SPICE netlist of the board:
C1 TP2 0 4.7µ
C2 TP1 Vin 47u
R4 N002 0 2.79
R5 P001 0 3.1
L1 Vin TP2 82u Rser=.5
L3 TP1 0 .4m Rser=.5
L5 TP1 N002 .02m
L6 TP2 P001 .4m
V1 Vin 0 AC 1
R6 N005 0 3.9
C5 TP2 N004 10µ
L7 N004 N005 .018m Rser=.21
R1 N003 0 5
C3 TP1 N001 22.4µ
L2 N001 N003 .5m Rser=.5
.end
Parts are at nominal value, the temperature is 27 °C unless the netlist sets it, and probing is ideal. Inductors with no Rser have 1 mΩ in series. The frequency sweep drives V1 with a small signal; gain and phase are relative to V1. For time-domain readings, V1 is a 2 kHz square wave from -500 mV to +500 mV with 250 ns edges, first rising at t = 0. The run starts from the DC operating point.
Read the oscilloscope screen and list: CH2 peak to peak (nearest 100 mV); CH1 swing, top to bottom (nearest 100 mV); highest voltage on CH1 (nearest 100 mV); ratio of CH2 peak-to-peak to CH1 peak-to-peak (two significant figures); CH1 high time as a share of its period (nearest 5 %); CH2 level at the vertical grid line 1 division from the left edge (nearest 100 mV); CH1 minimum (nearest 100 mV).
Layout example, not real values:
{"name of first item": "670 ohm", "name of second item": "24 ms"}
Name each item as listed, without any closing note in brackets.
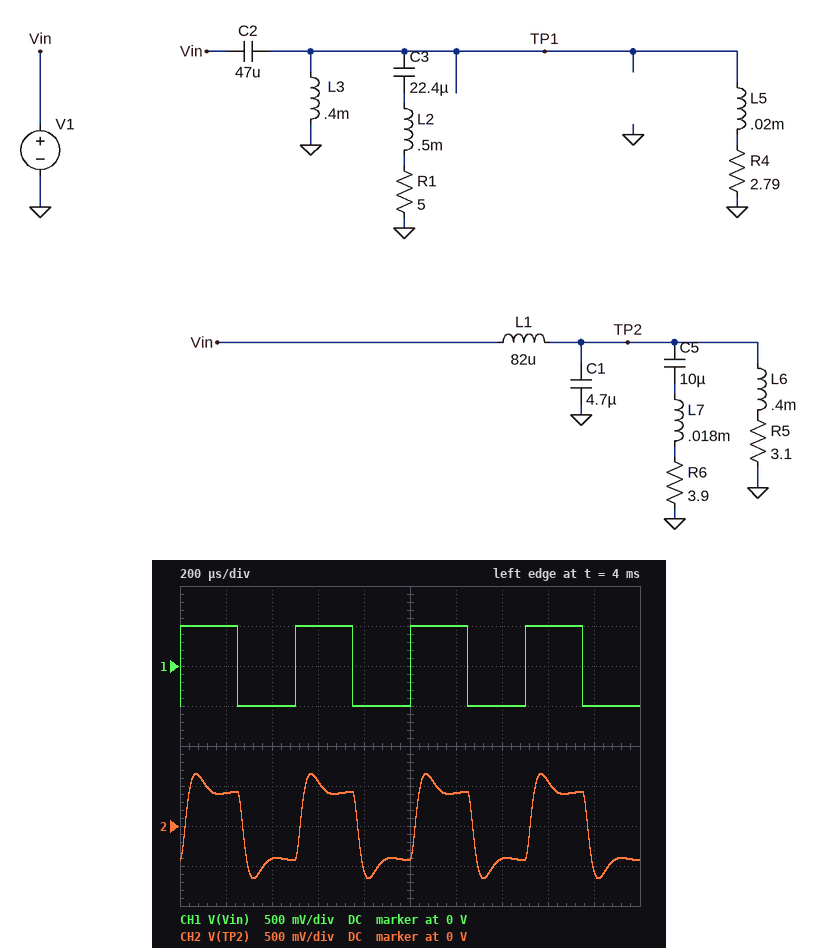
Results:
{"CH2 peak to peak": "1.3 V", "CH1 swing, top to bottom": "1.0 V", "highest voltage on CH1": "500 mV", "ratio of CH2 peak-to-peak to CH1 peak-to-peak": "1.3", "CH1 high time as a share of its period": "50 %", "CH2 level at the vertical grid line 1 division from the left edge": "400 mV", "CH1 minimum": "-500 mV"}
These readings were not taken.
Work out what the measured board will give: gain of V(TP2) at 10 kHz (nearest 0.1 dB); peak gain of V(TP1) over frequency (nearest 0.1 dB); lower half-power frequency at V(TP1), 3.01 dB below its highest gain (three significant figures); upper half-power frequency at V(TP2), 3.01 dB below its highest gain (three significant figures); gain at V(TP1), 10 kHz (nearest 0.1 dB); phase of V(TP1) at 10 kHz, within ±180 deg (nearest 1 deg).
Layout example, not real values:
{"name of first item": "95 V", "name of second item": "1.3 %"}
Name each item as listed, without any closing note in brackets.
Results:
{"gain of V(TP2) at 10 kHz": "-3.2 dB", "peak gain of V(TP1) over frequency": "1.4 dB", "lower half-power frequency at V(TP1), 3.01 dB below its highest gain": "1.68 kHz", "upper half-power frequency at V(TP2), 3.01 dB below its highest gain": "8.73 kHz", "gain at V(TP1), 10 kHz": "0.6 dB", "phase of V(TP1) at 10 kHz, within ±180 deg": "6 deg"}
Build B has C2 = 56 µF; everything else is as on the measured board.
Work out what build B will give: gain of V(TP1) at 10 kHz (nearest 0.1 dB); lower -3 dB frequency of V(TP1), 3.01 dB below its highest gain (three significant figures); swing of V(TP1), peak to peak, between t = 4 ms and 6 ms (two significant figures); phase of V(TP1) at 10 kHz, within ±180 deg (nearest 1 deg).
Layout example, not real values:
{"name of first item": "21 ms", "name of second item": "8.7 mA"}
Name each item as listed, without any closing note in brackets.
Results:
{"gain of V(TP1) at 10 kHz": "0.5 dB", "lower -3 dB frequency of V(TP1), 3.01 dB below its highest gain": "1.47 kHz", "swing of V(TP1), peak to peak, between t = 4 ms and 6 ms": "2.2 V", "phase of V(TP1) at 10 kHz, within ±180 deg": "5 deg"}
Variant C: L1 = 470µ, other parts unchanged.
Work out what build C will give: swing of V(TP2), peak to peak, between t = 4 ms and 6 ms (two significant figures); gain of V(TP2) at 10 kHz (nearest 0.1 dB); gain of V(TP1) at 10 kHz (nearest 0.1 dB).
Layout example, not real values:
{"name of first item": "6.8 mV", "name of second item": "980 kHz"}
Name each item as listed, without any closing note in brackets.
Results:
{"swing of V(TP2), peak to peak, between t = 4 ms and 6 ms": "910 mV", "gain of V(TP2) at 10 kHz": "-20.3 dB", "gain of V(TP1) at 10 kHz": "0.6 dB"}
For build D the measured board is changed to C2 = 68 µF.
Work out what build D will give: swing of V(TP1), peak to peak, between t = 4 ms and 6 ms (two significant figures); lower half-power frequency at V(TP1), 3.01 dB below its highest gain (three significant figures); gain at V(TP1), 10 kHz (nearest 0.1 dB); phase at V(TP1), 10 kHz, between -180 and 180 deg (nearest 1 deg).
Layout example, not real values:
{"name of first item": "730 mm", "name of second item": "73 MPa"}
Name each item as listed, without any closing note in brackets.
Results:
{"swing of V(TP1), peak to peak, between t = 4 ms and 6 ms": "2.1 V", "lower half-power frequency at V(TP1), 3.01 dB below its highest gain": "1.19 kHz", "gain at V(TP1), 10 kHz": "0.4 dB", "phase at V(TP1), 10 kHz, between -180 and 180 deg": "4 deg"}
